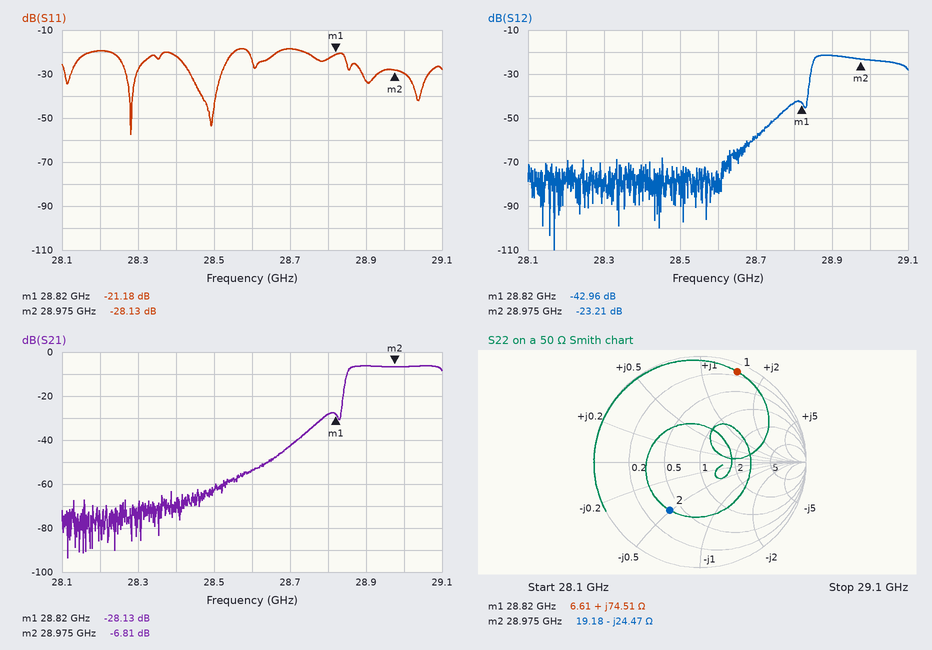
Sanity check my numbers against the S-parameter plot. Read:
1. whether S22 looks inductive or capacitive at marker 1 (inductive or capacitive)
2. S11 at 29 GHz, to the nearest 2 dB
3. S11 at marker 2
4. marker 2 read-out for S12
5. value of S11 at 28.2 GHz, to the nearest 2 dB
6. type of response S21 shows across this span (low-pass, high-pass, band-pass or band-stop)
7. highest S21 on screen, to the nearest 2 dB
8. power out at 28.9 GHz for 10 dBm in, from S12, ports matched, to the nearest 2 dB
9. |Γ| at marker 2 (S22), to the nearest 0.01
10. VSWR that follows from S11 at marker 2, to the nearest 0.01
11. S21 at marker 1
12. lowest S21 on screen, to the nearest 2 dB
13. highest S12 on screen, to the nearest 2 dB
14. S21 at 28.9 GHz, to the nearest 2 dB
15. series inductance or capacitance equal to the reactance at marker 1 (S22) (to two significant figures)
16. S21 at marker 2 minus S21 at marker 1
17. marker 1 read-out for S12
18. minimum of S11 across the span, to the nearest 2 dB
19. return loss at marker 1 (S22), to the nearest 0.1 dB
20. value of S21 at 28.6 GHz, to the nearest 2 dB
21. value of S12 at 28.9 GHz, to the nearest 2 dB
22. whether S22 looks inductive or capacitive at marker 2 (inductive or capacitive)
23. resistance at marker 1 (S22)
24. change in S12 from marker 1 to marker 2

inductive
-30 dB
-28.13 dB
-23.21 dB
-20 dB
high-pass
-6 dB
-12 dBm
0.54
1.08
-28.13 dB
-94 dB
-22 dB
-6 dB
410 pH
21.32 dB
-42.96 dB
-58 dB
0.7 dB
-54 dB
-22 dB
capacitive
6.61 Ω
19.75 dB
